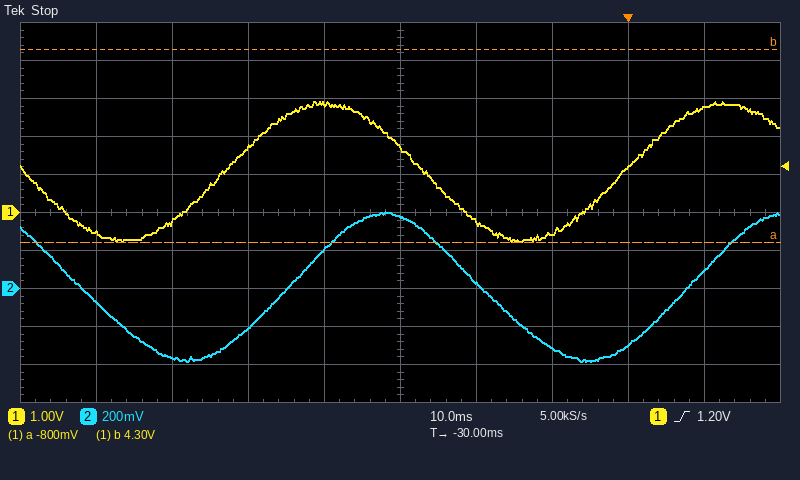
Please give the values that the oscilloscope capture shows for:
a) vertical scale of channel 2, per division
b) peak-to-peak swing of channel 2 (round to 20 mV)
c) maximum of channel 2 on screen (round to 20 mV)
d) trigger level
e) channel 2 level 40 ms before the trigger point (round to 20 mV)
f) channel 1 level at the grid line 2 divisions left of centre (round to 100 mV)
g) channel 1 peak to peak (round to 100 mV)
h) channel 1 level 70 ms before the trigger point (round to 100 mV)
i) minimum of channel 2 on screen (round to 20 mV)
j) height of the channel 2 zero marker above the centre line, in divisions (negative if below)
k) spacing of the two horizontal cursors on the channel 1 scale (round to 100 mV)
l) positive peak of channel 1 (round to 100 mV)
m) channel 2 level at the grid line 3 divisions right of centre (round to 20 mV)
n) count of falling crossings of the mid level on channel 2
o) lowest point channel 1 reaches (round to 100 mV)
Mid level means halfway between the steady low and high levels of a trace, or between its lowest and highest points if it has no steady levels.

200 mV
780 mV
400 mV
1.20 V
200 mV
1.7 V
3.7 V
-500 mV
-380 mV
-2.0 div
5.1 V
2.9 V
-300 mV
2
-800 mV
